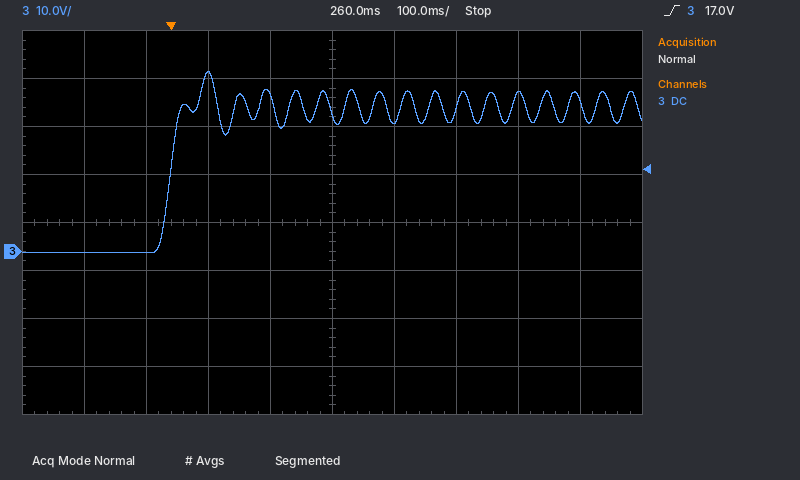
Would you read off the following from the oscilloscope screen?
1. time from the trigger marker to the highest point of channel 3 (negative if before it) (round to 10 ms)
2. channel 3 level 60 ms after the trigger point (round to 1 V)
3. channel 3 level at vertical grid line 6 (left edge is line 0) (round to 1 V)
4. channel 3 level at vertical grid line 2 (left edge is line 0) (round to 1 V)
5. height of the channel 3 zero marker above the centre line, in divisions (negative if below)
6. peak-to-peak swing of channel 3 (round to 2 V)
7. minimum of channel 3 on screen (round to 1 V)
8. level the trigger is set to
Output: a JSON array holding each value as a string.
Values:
["+60 ms", "37 V", "27 V", "0 V", "-0.6 div", "38 V", "0 V", "17.0 V"]
